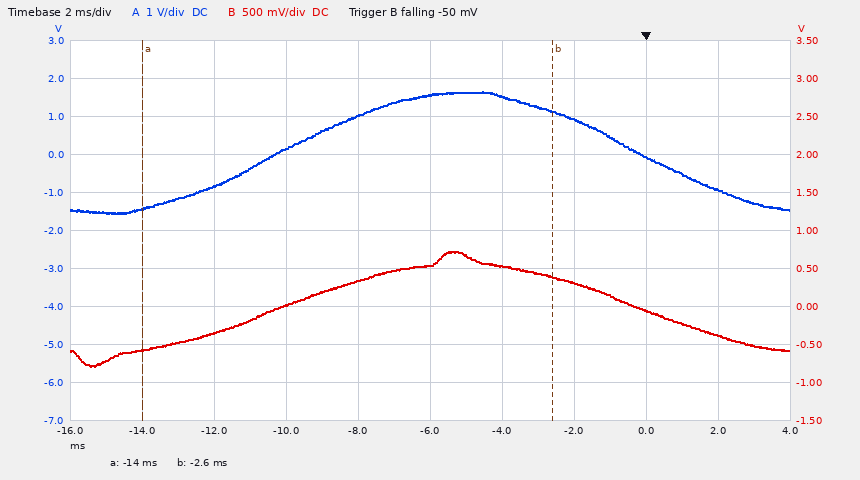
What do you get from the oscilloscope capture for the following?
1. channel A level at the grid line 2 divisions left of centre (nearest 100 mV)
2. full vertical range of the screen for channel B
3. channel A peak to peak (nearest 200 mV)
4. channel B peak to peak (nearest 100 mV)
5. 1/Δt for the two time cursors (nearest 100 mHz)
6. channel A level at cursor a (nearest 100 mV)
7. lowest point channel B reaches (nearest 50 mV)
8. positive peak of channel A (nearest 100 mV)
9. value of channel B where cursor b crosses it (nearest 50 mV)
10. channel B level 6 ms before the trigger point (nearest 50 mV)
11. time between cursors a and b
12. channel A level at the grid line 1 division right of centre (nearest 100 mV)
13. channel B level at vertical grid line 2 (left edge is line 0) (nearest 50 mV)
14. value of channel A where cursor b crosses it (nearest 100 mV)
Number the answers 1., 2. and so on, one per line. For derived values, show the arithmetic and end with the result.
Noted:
1. 200 mV
2. 5 V
3. 3.2 V
4. 1.50 V
5. 1 / 11.4 ms ≈ 87.7 Hz
6. -1.4 V
7. -800 mV
8. 1.7 V
9. 400 mV
10. 550 mV
11. -2.6 ms − (-14 ms) = 11.4 ms
12. 1.5 V
13. -350 mV
14. 1.1 V
